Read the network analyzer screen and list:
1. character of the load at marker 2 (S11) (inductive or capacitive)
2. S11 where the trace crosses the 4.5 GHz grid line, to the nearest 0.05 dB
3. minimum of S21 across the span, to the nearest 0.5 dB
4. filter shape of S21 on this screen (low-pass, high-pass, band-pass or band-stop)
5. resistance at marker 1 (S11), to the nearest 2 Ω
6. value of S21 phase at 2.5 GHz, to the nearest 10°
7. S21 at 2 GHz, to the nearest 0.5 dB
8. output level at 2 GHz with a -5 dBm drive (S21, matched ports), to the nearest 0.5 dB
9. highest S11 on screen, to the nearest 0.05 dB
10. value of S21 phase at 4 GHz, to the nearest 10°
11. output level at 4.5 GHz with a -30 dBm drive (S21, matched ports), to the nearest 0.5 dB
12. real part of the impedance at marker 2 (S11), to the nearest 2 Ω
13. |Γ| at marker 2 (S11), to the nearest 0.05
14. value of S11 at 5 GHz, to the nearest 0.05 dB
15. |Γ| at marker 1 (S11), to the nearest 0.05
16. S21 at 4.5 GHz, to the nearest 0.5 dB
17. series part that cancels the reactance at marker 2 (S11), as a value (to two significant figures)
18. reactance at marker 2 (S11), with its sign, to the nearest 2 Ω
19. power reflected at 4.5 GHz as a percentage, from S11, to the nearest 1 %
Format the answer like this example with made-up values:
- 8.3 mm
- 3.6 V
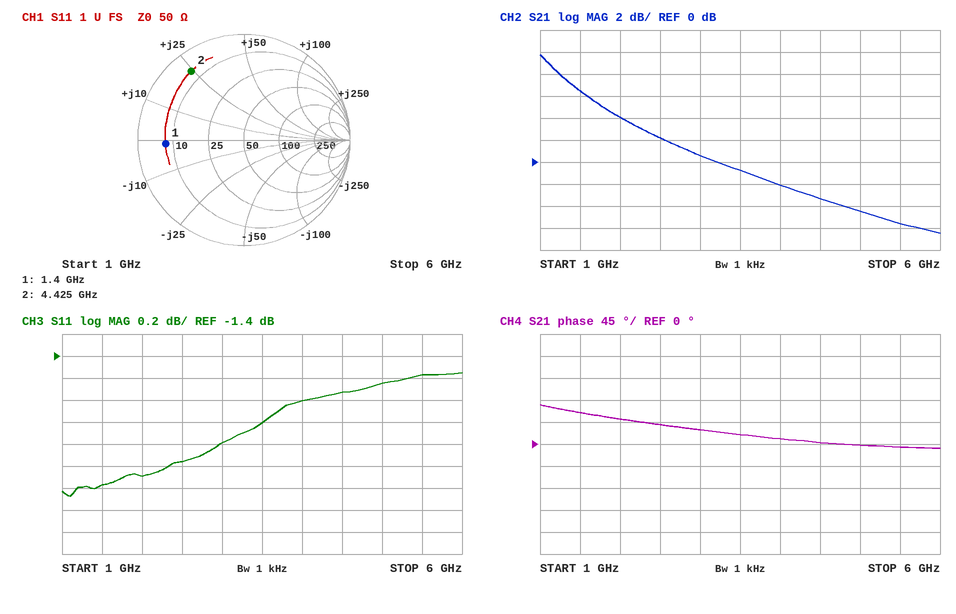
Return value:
- inductive
- -1.75 dB
- -6.5 dB
- low-pass
- 8 Ω
- 40°
- 4.0 dB
- -1.0 dBm
- -1.55 dB
- 10°
- -33.5 dBm
- 6 Ω
- 0.80
- -1.65 dB
- 0.75
- -3.5 dB
- 1.5 pF
- +24 Ω
- 67 %
